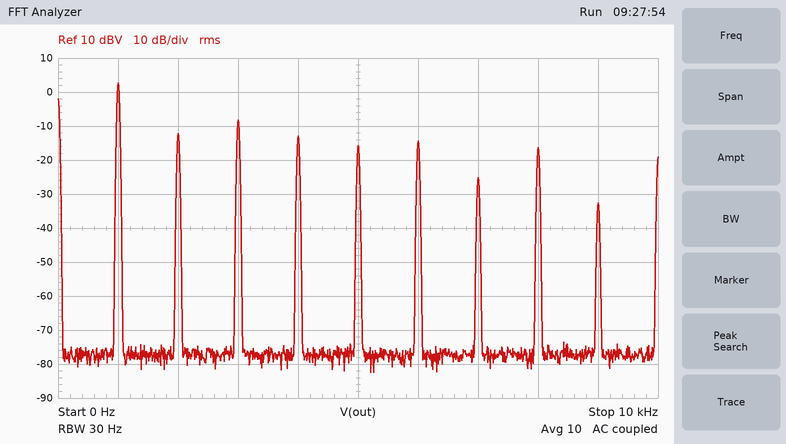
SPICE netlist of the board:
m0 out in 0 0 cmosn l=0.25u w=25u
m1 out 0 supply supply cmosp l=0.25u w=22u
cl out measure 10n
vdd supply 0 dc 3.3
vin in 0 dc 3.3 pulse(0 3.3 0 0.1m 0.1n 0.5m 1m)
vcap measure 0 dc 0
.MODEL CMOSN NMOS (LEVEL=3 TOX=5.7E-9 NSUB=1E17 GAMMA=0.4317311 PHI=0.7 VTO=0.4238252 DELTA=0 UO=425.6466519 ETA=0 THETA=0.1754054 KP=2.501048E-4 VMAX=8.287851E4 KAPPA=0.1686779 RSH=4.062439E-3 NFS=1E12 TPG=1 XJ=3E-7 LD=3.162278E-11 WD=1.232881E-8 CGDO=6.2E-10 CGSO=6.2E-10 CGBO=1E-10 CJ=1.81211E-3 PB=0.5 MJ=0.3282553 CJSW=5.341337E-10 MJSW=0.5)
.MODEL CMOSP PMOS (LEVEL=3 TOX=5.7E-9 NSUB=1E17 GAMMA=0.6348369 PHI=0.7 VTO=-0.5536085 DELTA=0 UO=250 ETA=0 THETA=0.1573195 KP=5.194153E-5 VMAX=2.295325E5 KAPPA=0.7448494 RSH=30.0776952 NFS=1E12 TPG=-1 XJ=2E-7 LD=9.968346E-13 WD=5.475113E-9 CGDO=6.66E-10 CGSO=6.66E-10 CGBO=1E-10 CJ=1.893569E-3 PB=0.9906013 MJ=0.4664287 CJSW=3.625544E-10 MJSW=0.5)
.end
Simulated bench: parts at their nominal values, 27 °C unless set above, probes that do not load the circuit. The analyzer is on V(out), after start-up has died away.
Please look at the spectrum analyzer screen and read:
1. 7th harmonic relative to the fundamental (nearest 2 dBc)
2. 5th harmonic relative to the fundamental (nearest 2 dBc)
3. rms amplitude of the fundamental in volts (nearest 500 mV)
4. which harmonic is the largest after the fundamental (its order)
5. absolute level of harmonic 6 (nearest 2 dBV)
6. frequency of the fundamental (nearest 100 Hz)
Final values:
-28 dBc
-18 dBc
1.5 V
3
-14 dBV
1.0 kHz
